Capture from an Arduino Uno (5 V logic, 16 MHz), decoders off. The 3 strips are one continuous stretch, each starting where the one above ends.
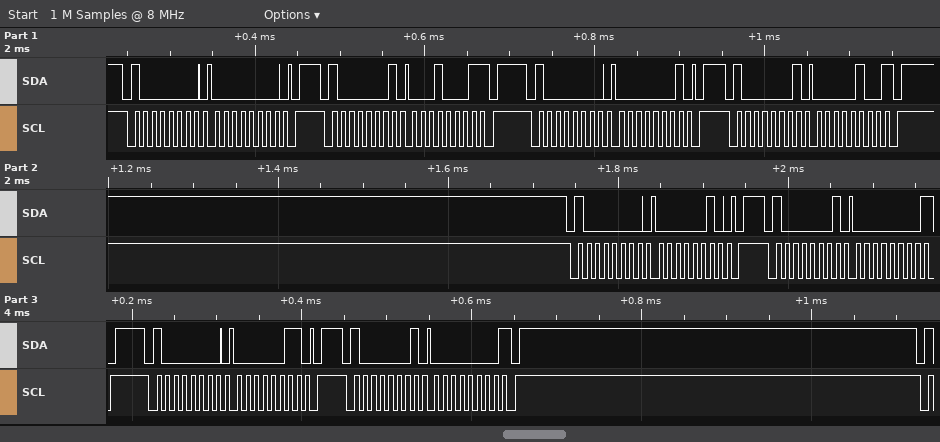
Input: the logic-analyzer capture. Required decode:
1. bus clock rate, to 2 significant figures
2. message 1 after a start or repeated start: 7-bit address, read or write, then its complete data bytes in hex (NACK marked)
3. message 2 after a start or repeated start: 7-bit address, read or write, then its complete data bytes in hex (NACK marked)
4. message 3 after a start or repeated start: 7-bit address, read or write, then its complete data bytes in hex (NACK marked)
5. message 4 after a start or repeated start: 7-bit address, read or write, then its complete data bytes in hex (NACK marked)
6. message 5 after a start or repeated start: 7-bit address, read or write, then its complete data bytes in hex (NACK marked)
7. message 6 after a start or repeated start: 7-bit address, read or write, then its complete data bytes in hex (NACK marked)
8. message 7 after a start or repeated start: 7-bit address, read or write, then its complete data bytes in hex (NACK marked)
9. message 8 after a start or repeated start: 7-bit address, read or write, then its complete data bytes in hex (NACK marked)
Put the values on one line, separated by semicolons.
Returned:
100 kHz; 0x40 write: 00; 0x40 read: 11 NACK; 0x40 write: 01; 0x40 read: 04 NACK; 0x40 write: 02; 0x40 read: 00 NACK; 0x40 write: 03; 0x40 read: 00 NACK
